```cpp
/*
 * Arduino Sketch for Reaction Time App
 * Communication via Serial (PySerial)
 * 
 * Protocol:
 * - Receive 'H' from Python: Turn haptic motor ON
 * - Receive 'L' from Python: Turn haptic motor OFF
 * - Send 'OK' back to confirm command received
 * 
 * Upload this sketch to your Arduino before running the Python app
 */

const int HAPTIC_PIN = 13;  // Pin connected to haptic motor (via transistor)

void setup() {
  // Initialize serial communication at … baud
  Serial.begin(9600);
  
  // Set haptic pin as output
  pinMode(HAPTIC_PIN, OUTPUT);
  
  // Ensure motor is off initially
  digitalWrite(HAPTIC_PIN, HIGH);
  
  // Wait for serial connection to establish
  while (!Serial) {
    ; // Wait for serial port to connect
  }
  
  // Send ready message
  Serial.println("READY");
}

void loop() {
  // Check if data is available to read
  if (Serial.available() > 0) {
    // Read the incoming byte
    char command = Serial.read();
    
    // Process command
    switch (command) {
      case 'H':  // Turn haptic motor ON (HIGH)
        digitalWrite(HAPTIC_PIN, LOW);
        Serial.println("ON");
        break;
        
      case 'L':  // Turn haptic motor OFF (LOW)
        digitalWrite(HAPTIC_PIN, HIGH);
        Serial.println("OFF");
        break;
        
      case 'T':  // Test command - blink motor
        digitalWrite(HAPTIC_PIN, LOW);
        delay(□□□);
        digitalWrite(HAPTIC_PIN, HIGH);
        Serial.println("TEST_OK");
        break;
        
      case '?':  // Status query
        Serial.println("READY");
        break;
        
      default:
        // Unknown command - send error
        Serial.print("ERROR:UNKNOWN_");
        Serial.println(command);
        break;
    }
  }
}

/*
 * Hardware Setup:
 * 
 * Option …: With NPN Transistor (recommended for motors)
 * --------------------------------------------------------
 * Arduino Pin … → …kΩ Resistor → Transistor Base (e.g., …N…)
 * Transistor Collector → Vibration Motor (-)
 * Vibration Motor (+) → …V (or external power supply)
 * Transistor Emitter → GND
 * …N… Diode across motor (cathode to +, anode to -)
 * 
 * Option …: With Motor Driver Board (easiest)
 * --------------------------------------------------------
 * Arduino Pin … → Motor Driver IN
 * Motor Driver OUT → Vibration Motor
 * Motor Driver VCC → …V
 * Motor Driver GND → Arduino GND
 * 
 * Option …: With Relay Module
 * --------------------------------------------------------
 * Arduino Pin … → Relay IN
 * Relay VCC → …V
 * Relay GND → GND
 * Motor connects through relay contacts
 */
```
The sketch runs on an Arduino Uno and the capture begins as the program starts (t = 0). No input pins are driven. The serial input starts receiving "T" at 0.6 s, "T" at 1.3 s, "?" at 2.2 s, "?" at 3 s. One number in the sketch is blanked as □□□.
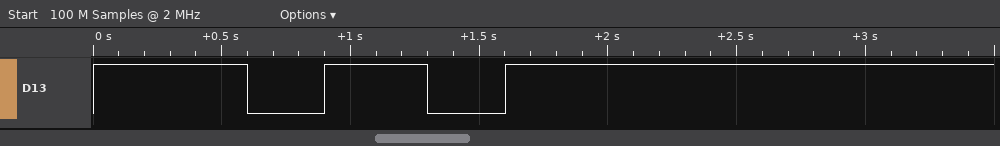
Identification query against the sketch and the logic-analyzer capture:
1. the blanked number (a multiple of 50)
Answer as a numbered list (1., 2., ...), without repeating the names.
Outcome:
1. 300
